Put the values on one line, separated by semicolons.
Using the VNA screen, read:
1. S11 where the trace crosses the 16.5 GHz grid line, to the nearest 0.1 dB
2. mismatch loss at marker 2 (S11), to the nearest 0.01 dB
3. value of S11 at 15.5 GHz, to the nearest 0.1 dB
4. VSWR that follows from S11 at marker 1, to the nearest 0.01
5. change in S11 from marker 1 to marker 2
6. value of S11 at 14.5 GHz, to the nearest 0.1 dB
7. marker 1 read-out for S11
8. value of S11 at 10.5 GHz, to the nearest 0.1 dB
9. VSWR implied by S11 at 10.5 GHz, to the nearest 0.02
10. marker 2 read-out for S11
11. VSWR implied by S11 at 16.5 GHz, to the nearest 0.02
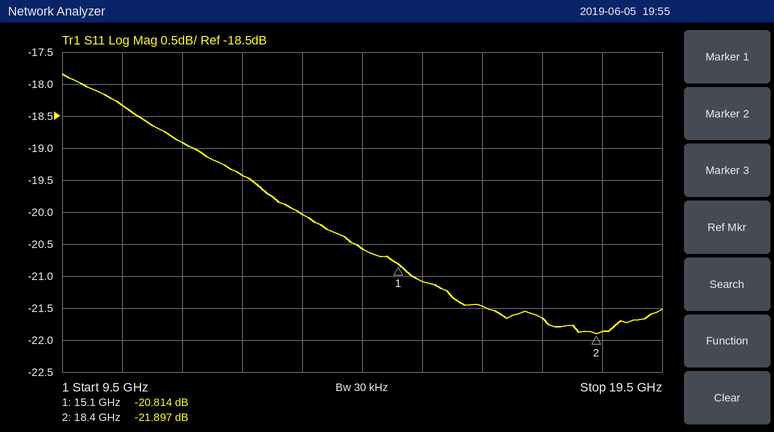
-21.5 dB; 0.03 dB; -21.1 dB; 1.20; -1.083 dB; -20.6 dB; -20.814 dB; -18.3 dB; 1.28; -21.897 dB; 1.18
